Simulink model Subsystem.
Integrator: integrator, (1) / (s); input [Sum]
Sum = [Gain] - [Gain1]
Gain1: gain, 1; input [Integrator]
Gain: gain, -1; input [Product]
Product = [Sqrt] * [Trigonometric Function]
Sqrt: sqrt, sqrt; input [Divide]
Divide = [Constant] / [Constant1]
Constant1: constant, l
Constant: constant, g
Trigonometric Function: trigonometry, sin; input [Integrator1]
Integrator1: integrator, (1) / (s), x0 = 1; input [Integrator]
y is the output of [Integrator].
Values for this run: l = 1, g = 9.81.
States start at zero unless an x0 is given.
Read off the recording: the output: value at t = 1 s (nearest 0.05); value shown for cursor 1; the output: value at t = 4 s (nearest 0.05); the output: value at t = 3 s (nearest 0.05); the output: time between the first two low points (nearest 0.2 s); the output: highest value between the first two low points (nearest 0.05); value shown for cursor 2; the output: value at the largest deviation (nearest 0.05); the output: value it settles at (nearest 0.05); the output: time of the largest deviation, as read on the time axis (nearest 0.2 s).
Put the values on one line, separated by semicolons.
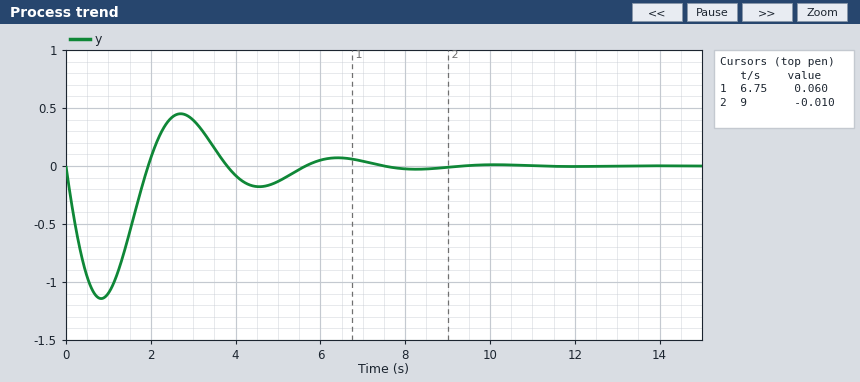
-1.10; 0.060; -0.10; 0.40; 3.8 s; 0.45; -0.010; -1.15; 0.00; 0.8 s
